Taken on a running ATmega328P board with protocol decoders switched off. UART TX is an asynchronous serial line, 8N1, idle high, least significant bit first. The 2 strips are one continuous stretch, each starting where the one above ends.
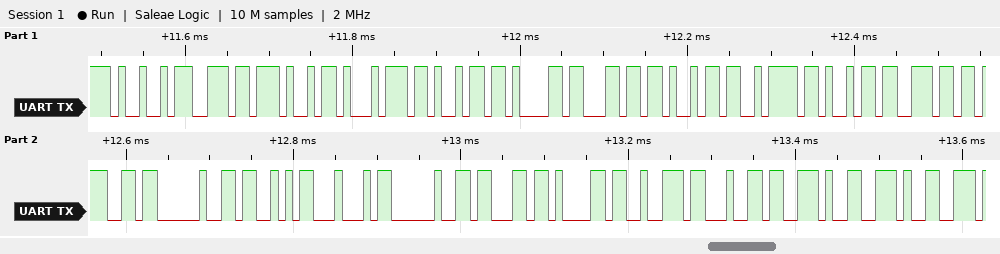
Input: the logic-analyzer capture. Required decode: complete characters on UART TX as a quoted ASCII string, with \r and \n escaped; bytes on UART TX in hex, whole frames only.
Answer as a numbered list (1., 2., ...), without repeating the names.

1. "Initializing SD card.."
2. 49 6E 69 74 69 61 6C 69 7A 69 6E 67 20 53 44 20 63 61 72 64 2E 2E
